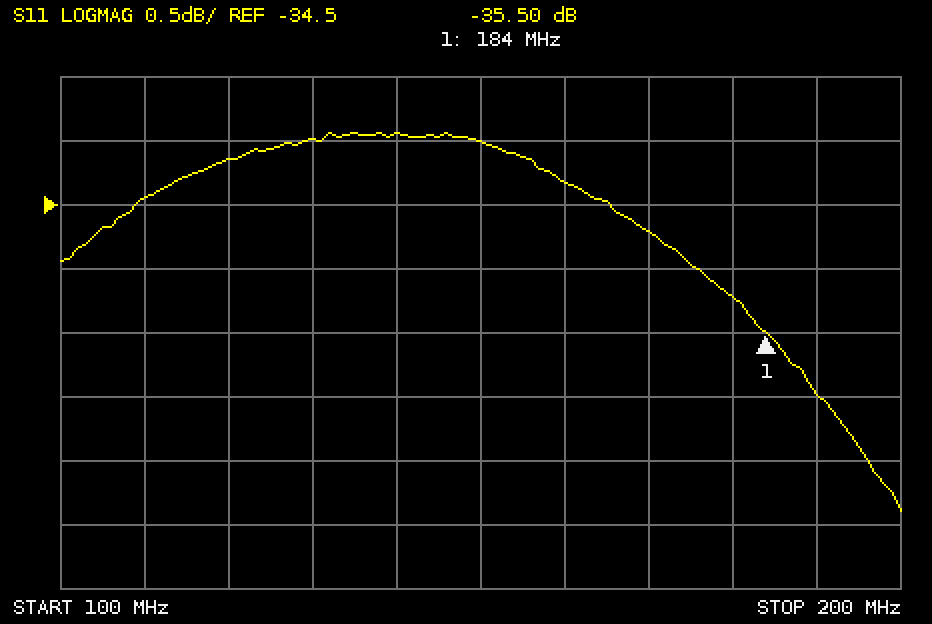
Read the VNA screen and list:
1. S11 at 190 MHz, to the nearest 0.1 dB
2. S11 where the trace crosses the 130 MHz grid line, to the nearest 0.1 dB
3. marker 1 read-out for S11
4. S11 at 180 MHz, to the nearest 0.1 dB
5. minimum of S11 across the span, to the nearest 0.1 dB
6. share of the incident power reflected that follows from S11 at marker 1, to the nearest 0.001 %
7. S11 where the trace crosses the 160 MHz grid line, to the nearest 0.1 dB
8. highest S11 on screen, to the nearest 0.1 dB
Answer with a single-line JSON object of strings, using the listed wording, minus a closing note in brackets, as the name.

{"S11 at 190 MHz, to the nearest 0.1 dB": "-36.0 dB", "S11 where the trace crosses the 130 MHz grid line, to the nearest 0.1 dB": "-34.0 dB", "marker 1 read-out for S11": "-35.50 dB", "S11 at 180 MHz, to the nearest 0.1 dB": "-35.2 dB", "minimum of S11 across the span, to the nearest 0.1 dB": "-36.9 dB", "share of the incident power reflected that follows from S11 at marker 1, to the nearest 0.001 %": "0.028 %", "S11 where the trace crosses the 160 MHz grid line, to the nearest 0.1 dB": "-34.3 dB", "highest S11 on screen, to the nearest 0.1 dB": "-33.9 dB"}
